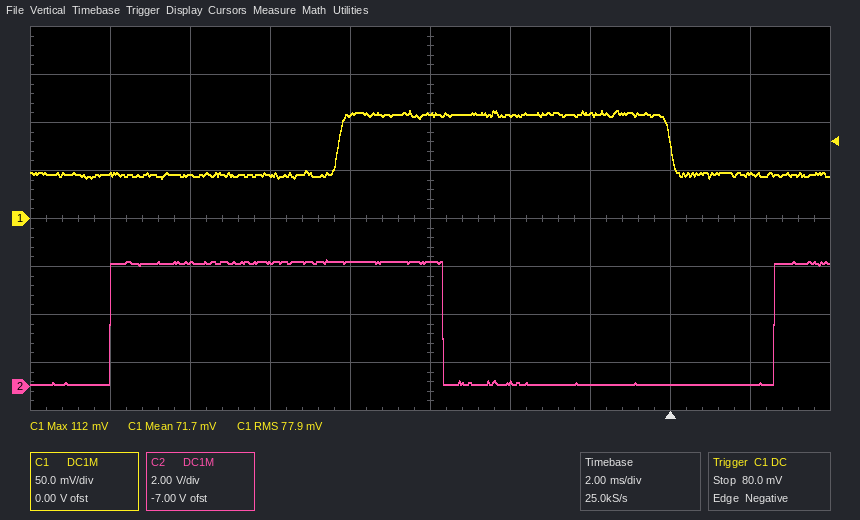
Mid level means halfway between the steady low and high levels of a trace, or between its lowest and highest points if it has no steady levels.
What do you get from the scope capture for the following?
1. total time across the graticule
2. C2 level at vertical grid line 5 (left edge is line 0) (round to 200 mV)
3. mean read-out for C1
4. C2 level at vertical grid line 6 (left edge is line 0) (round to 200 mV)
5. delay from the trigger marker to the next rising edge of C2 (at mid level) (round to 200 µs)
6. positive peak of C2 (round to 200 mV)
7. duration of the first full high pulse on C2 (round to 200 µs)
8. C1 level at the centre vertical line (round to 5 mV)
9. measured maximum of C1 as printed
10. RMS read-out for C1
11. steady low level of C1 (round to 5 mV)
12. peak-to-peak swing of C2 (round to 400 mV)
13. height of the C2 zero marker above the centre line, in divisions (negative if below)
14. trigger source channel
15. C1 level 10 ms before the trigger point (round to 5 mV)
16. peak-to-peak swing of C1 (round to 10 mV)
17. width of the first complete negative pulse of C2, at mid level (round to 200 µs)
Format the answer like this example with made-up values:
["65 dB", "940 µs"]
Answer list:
["20 ms", "5.2 V", "71.7 mV", "200 mV", "2.6 ms", "5.2 V", "8.4 ms", "110 mV", "112 mV", "77.9 mV", "45 mV", "5.2 V", "-3.5 div", "C1", "45 mV", "70 mV", "8.2 ms"]
